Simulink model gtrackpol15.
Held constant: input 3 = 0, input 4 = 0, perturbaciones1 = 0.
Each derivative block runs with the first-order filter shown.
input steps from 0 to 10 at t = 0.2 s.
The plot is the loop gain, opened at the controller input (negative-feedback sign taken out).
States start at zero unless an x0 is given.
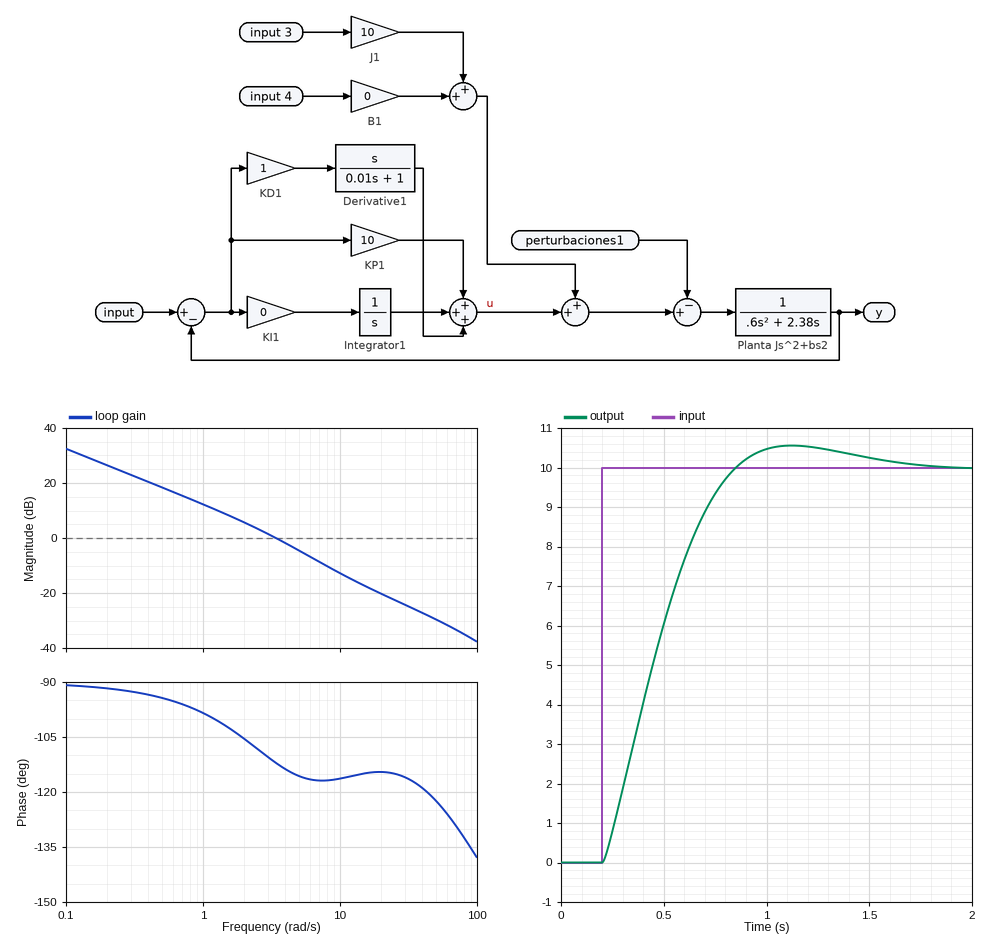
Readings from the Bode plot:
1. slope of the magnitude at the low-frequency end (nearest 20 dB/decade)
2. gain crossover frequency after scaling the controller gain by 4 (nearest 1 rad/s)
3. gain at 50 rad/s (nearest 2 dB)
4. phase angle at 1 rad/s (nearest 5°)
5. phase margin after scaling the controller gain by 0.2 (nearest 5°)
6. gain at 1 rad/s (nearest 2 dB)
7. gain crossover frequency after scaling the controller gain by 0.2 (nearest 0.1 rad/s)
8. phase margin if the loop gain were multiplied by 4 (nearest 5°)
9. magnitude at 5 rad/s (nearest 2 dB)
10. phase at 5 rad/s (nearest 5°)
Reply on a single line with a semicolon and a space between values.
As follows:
-20 dB/decade; 9 rad/s; -30 dB; -100°; 85°; 12 dB; 0.8 rad/s; 65°; -4 dB; -115°
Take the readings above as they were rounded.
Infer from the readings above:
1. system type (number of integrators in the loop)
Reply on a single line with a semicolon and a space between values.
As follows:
1
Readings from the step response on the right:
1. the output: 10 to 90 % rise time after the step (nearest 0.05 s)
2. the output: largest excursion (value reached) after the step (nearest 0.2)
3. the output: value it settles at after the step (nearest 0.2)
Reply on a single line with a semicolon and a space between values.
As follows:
0.45 s; 10.6; 10.0
